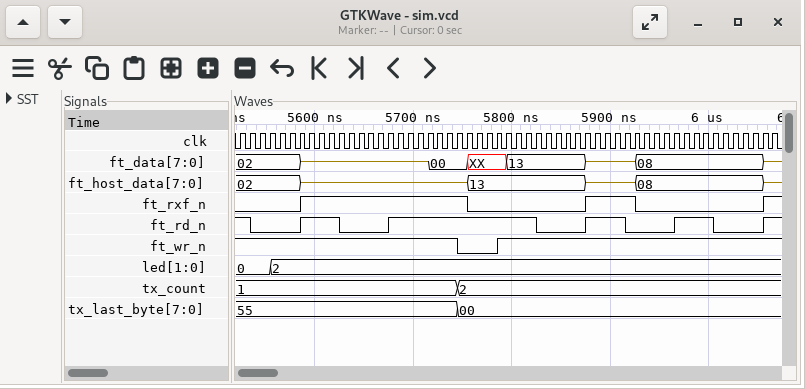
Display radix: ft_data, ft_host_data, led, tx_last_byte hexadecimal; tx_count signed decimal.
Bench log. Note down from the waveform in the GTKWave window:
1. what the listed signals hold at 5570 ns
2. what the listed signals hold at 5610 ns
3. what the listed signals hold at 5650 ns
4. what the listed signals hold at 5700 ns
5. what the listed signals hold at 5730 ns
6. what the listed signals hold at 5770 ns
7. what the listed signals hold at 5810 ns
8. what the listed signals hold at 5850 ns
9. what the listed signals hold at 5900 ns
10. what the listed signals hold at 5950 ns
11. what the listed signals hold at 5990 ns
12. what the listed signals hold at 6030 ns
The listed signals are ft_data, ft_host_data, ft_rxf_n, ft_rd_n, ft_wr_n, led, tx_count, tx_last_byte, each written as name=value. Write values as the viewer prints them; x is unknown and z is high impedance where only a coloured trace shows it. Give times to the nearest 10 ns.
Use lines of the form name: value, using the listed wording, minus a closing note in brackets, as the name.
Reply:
what the listed signals hold at 5570 ns: ft_data=02, ft_host_data=02, ft_rxf_n=0, ft_rd_n=0, ft_wr_n=1, led=2, tx_count=1, tx_last_byte=55
what the listed signals hold at 5610 ns: ft_data=z, ft_host_data=z, ft_rxf_n=1, ft_rd_n=1, ft_wr_n=1, led=2, tx_count=1, tx_last_byte=55
what the listed signals hold at 5650 ns: ft_data=z, ft_host_data=z, ft_rxf_n=1, ft_rd_n=0, ft_wr_n=1, led=2, tx_count=1, tx_last_byte=55
what the listed signals hold at 5700 ns: ft_data=z, ft_host_data=z, ft_rxf_n=1, ft_rd_n=1, ft_wr_n=1, led=2, tx_count=1, tx_last_byte=55
what the listed signals hold at 5730 ns: ft_data=00, ft_host_data=z, ft_rxf_n=1, ft_rd_n=1, ft_wr_n=1, led=2, tx_count=1, tx_last_byte=55
what the listed signals hold at 5770 ns: ft_data=XX, ft_host_data=13, ft_rxf_n=0, ft_rd_n=1, ft_wr_n=0, led=2, tx_count=2, tx_last_byte=00
what the listed signals hold at 5810 ns: ft_data=13, ft_host_data=13, ft_rxf_n=0, ft_rd_n=1, ft_wr_n=1, led=2, tx_count=2, tx_last_byte=00
what the listed signals hold at 5850 ns: ft_data=13, ft_host_data=13, ft_rxf_n=0, ft_rd_n=0, ft_wr_n=1, led=2, tx_count=2, tx_last_byte=00
what the listed signals hold at 5900 ns: ft_data=z, ft_host_data=z, ft_rxf_n=1, ft_rd_n=1, ft_wr_n=1, led=2, tx_count=2, tx_last_byte=00
what the listed signals hold at 5950 ns: ft_data=08, ft_host_data=08, ft_rxf_n=0, ft_rd_n=0, ft_wr_n=1, led=2, tx_count=2, tx_last_byte=00
what the listed signals hold at 5990 ns: ft_data=08, ft_host_data=08, ft_rxf_n=0, ft_rd_n=1, ft_wr_n=1, led=2, tx_count=2, tx_last_byte=00
what the listed signals hold at 6030 ns: ft_data=08, ft_host_data=08, ft_rxf_n=0, ft_rd_n=0, ft_wr_n=1, led=2, tx_count=2, tx_last_byte=00
